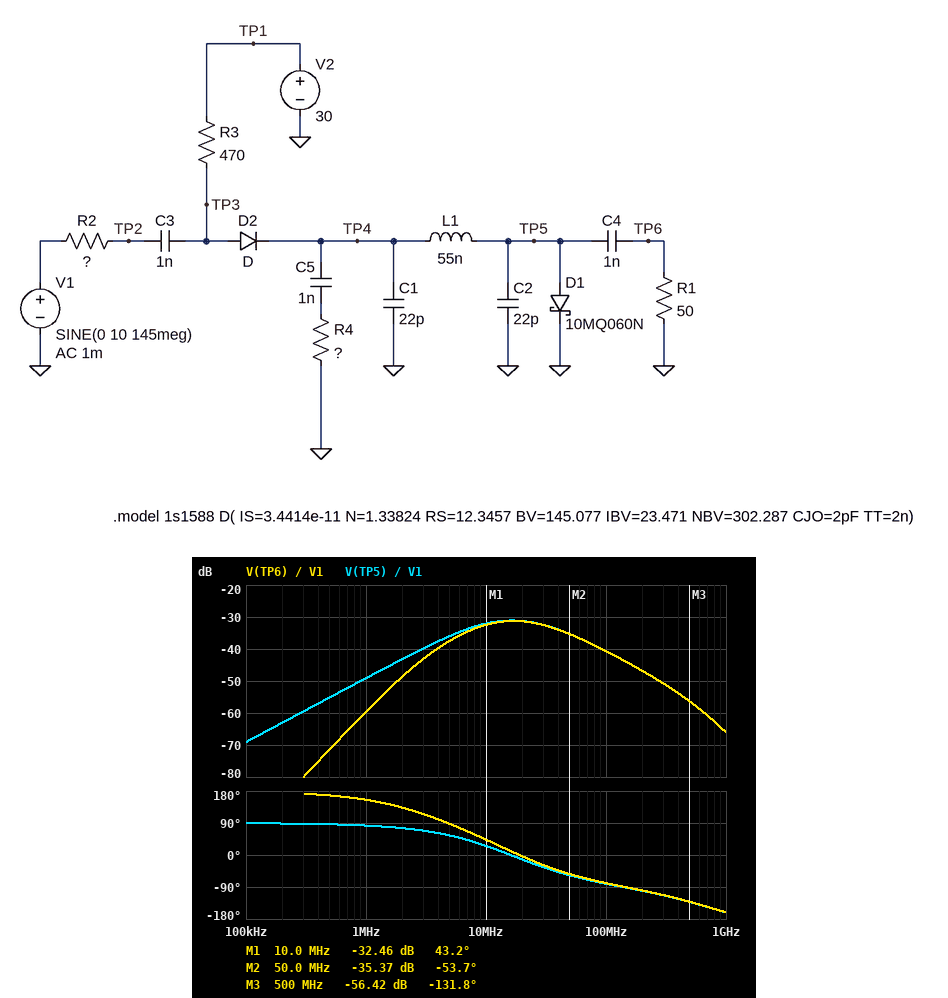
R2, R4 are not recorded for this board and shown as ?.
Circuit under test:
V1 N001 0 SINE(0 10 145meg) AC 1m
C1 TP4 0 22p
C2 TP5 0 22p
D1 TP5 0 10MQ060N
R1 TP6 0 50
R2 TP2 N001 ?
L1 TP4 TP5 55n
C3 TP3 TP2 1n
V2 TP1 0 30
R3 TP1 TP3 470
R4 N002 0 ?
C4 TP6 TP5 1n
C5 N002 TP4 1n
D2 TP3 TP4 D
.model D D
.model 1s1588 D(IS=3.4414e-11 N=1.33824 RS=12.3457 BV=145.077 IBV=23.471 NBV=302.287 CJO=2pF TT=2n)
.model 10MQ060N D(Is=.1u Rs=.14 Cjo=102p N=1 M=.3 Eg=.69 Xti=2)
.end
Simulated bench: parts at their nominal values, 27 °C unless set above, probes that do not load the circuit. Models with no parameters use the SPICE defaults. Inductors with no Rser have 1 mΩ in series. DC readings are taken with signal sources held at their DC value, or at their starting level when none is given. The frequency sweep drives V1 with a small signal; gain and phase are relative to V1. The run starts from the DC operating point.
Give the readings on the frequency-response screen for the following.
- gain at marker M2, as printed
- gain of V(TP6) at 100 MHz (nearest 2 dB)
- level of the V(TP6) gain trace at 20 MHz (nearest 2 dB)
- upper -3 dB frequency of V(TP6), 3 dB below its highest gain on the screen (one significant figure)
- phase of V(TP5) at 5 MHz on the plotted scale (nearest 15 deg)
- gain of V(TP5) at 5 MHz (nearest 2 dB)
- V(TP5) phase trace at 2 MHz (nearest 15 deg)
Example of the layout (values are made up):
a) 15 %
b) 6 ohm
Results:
a) -35.37 dB
b) -40 dB
c) -32 dB
d) 40 MHz
e) 60 deg
f) -36 dB
g) 75 deg
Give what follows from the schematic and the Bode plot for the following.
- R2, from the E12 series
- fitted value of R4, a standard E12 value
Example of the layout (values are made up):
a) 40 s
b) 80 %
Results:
a) 18 Ω
b) 27 Ω
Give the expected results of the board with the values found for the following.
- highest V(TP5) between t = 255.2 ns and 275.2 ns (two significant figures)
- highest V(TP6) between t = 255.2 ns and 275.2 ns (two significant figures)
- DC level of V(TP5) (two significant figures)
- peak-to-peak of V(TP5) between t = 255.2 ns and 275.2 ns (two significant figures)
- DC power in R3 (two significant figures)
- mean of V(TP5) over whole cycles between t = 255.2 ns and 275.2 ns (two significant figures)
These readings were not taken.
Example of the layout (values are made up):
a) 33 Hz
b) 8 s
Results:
a) 380 mV
b) 33 mV
c) 350 mV
d) 77 mV
e) 1.8 W
f) 350 mV
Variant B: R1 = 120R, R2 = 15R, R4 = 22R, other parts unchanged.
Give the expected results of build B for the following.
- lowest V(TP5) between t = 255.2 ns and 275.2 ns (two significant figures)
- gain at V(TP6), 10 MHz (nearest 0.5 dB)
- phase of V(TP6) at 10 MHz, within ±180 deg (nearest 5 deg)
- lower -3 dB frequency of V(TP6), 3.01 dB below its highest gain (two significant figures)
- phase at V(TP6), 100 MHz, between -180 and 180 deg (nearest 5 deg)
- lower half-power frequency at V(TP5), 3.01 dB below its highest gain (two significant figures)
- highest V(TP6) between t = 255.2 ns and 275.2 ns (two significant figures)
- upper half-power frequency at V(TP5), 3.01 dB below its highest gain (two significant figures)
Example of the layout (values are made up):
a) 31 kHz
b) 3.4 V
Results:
a) 320 mV
b) -31.0 dB
c) 35 deg
d) 7.4 MHz
e) -80 deg
f) 7.3 MHz
g) 26 mV
h) 36 MHz
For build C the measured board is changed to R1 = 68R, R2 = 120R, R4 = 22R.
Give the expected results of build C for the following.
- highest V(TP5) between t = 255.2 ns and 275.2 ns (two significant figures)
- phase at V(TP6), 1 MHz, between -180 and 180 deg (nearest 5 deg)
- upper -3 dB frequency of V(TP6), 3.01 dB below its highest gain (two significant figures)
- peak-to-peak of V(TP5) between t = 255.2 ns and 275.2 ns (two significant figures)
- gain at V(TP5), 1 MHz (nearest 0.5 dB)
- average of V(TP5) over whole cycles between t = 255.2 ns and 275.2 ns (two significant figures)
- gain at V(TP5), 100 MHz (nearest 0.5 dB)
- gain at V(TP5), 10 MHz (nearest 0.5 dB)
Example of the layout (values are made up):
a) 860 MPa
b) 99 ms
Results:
a) 370 mV
b) 120 deg
c) 60 MHz
d) 34 mV
e) -51.0 dB
f) 350 mV
g) -52.5 dB
h) -46.5 dB
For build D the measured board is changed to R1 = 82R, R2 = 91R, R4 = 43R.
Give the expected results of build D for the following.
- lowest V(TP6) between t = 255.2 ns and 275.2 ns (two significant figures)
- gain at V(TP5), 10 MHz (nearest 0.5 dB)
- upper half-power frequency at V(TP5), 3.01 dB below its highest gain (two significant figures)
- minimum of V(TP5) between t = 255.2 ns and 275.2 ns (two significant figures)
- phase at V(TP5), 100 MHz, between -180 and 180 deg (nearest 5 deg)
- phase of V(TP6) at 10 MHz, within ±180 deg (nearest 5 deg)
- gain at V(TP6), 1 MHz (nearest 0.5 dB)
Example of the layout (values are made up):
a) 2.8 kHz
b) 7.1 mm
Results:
a) -57 mV
b) -44.5 dB
c) 110 MHz
d) 290 mV
e) -70 deg
f) 15 deg
g) -57.0 dB
